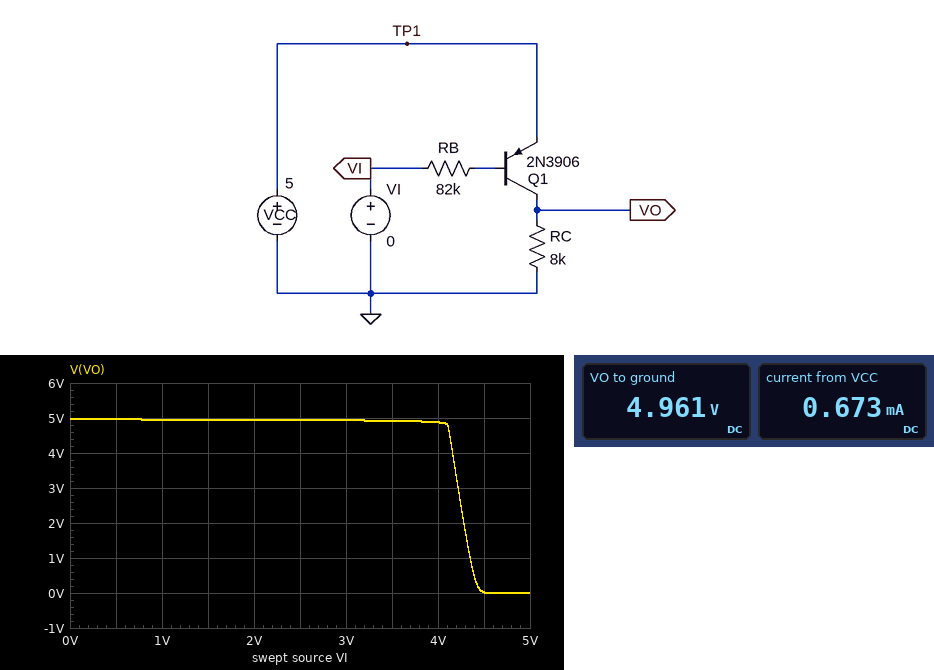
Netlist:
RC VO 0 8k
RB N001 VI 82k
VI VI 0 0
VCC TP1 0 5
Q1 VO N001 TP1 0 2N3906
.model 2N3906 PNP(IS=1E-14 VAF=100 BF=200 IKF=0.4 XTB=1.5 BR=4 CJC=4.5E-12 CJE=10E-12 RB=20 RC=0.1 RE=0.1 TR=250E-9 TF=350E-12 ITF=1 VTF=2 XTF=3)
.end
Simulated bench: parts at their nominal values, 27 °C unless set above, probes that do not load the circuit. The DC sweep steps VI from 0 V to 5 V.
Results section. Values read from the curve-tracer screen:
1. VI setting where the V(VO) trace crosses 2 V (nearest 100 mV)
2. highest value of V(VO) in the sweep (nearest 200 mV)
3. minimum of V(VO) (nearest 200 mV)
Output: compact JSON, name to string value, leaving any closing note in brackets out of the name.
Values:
{"VI setting where the V(VO) trace crosses 2 V": "4.3 V", "highest value of V(VO) in the sweep": "5.0 V", "minimum of V(VO)": "0 V"}
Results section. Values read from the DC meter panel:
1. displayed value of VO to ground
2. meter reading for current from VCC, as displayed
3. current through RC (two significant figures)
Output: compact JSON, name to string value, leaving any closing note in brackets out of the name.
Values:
{"displayed value of VO to ground": "4.961 V", "meter reading for current from VCC, as displayed": "0.673 mA", "current through RC": "620 µA"}
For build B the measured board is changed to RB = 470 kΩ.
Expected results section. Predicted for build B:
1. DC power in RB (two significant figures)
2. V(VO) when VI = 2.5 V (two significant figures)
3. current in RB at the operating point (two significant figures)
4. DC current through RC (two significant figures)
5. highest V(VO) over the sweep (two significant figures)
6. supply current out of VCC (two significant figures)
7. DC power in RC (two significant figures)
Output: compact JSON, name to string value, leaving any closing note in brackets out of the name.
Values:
{"DC power in RB": "40 µW", "V(VO) when VI = 2.5 V": "4.9 V", "current in RB at the operating point": "9.3 µA", "DC current through RC": "610 µA", "highest V(VO) over the sweep": "4.9 V", "supply current out of VCC": "620 µA", "DC power in RC": "3.0 mW"}
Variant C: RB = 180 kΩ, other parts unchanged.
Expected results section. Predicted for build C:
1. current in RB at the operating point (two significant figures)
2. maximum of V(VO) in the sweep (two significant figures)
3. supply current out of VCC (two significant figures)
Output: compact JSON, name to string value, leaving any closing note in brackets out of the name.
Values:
{"current in RB at the operating point": "24 µA", "maximum of V(VO) in the sweep": "4.9 V", "supply current out of VCC": "640 µA"}
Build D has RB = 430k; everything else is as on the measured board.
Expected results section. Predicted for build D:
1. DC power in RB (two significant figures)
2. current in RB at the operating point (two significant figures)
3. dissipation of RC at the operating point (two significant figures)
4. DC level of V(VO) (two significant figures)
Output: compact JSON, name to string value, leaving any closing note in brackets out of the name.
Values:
{"DC power in RB": "44 µW", "current in RB at the operating point": "10 µA", "dissipation of RC at the operating point": "3.0 mW", "DC level of V(VO)": "4.9 V"}
